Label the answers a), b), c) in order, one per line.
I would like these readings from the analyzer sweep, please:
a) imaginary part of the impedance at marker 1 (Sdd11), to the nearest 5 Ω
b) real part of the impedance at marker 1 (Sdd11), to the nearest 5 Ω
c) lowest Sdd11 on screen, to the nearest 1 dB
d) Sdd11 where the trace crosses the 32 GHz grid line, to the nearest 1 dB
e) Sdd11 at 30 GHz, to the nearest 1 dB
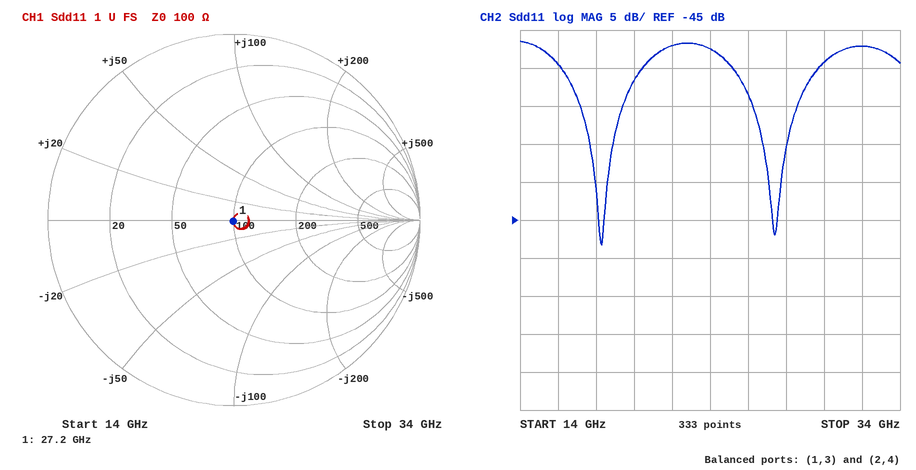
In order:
a) 0 Ω
b) 100 Ω
c) -48 dB
d) -22 dB
e) -24 dB
